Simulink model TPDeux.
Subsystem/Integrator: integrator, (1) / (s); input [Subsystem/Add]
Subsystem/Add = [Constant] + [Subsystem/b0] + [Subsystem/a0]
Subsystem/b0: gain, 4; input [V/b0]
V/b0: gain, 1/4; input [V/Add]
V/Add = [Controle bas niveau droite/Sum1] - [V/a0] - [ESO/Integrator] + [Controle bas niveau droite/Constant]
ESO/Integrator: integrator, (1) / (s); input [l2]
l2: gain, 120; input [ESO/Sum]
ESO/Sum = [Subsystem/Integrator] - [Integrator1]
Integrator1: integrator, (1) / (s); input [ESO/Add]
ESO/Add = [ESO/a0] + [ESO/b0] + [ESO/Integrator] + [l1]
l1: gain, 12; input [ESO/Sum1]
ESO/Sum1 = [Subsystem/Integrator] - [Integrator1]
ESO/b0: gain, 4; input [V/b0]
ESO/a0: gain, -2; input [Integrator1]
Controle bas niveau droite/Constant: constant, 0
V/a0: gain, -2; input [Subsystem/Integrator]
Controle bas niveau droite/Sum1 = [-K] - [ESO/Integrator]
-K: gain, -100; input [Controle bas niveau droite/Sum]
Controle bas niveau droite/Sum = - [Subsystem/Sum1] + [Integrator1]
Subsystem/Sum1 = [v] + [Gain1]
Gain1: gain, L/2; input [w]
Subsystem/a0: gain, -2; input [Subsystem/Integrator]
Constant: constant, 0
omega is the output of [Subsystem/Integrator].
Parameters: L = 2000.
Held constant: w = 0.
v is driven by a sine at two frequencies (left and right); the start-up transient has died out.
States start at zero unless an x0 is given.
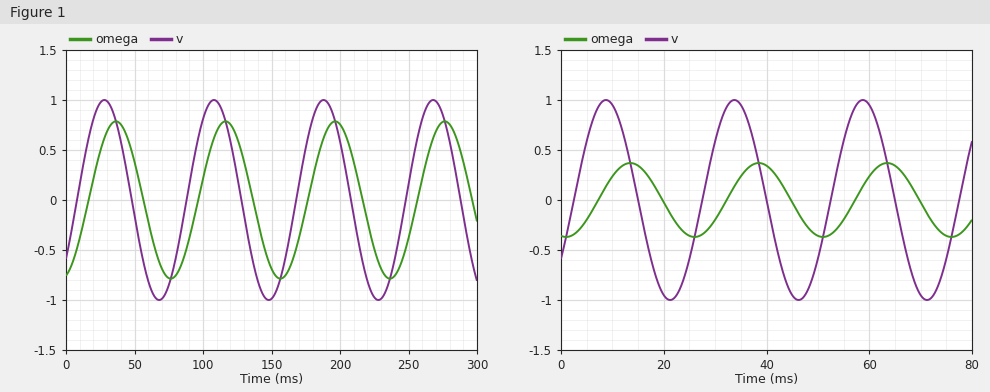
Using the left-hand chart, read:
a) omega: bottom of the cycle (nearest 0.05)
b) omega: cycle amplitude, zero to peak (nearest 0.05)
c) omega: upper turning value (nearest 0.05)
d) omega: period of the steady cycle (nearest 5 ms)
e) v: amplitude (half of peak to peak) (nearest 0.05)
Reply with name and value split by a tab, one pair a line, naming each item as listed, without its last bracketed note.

omega: bottom of the cycle	-0.80
omega: cycle amplitude, zero to peak	0.80
omega: upper turning value	0.80
omega: period of the steady cycle	80 ms
v: amplitude (half of peak to peak)	1.00
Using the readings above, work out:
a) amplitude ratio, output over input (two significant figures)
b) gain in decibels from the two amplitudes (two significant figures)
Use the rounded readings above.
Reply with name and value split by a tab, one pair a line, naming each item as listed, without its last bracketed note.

amplitude ratio, output over input	0.80
gain in decibels from the two amplitudes	-1.9 dB
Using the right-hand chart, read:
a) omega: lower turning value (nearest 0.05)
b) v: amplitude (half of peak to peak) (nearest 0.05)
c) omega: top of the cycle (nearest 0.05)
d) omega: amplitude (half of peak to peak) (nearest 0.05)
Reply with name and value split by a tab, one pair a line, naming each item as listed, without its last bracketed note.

omega: lower turning value	-0.35
v: amplitude (half of peak to peak)	1.00
omega: top of the cycle	0.35
omega: amplitude (half of peak to peak)	0.35
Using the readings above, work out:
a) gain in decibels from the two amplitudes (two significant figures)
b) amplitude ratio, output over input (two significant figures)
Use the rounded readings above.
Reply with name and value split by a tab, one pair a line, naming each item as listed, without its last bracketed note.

gain in decibels from the two amplitudes	-9.1 dB
amplitude ratio, output over input	0.35
